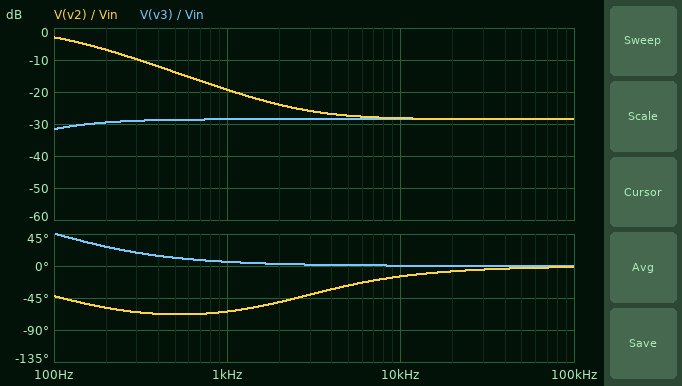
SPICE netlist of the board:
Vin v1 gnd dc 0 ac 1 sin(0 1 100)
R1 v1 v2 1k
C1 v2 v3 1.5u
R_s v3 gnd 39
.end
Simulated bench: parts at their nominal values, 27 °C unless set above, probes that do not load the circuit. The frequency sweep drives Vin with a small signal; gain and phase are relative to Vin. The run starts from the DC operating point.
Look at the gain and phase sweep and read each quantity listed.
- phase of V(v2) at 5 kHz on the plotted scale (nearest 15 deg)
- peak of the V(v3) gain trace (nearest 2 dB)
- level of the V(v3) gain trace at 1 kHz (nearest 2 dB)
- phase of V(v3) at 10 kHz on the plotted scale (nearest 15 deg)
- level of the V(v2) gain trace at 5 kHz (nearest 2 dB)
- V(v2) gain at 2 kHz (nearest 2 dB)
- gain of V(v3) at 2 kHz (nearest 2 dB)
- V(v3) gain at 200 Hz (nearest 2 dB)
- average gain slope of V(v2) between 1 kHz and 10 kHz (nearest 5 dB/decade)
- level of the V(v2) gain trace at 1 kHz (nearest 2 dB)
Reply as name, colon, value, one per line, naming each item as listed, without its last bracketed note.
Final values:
phase of V(v2) at 5 kHz on the plotted scale: -30 deg
peak of the V(v3) gain trace: -28 dB
level of the V(v3) gain trace at 1 kHz: -28 dB
phase of V(v3) at 10 kHz on the plotted scale: 0 deg
level of the V(v2) gain trace at 5 kHz: -28 dB
V(v2) gain at 2 kHz: -24 dB
gain of V(v3) at 2 kHz: -28 dB
V(v3) gain at 200 Hz: -30 dB
average gain slope of V(v2) between 1 kHz and 10 kHz: -10 dB/decade
level of the V(v2) gain trace at 1 kHz: -20 dB
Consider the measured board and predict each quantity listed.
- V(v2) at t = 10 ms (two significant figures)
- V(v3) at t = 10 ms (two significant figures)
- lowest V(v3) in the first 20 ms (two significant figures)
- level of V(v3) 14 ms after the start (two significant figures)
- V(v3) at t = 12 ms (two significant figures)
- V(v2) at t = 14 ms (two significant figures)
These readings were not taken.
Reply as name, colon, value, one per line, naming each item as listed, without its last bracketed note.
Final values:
V(v2) at t = 10 ms: -480 mV
V(v3) at t = 10 ms: 19 mV
lowest V(v3) in the first 20 ms: -27 mV
level of V(v3) 14 ms after the start: -4.4 mV
V(v3) at t = 12 ms: 23 mV
V(v2) at t = 14 ms: 700 mV
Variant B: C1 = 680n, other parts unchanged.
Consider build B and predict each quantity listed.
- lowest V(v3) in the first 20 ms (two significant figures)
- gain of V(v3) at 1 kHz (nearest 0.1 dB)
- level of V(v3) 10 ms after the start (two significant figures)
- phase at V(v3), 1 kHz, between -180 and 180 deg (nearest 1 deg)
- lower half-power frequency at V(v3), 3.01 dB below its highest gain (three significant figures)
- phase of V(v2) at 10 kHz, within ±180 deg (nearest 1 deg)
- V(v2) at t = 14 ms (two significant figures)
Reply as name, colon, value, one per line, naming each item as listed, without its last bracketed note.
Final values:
lowest V(v3) in the first 20 ms: -15 mV
gain of V(v3) at 1 kHz: -28.7 dB
level of V(v3) 10 ms after the start: 14 mV
phase at V(v3), 1 kHz, between -180 and 180 deg: 13 deg
lower half-power frequency at V(v3), 3.01 dB below its highest gain: 225 Hz
phase of V(v2) at 10 kHz, within ±180 deg: -30 deg
V(v2) at t = 14 ms: 780 mV
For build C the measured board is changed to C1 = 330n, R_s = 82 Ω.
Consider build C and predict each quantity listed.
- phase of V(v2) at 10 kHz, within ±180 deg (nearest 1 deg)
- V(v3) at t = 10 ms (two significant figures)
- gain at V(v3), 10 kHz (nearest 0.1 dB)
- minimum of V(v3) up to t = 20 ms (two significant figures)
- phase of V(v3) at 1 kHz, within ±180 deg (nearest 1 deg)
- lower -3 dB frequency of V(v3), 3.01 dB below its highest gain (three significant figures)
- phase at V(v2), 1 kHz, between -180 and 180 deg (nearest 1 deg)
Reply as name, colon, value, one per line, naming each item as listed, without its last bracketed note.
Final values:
phase of V(v2) at 10 kHz, within ±180 deg: -28 deg
V(v3) at t = 10 ms: 16 mV
gain at V(v3), 10 kHz: -22.4 dB
minimum of V(v3) up to t = 20 ms: -17 mV
phase of V(v3) at 1 kHz, within ±180 deg: 24 deg
lower -3 dB frequency of V(v3), 3.01 dB below its highest gain: 446 Hz
phase at V(v2), 1 kHz, between -180 and 180 deg: -56 deg
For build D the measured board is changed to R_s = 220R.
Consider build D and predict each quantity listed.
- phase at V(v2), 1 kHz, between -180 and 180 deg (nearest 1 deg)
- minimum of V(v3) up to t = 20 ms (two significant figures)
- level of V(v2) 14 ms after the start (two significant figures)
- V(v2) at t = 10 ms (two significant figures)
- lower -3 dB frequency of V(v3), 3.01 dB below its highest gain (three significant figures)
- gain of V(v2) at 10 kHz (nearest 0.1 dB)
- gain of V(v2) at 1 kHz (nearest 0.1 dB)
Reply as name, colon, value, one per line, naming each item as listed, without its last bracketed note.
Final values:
phase at V(v2), 1 kHz, between -180 and 180 deg: -21 deg
minimum of V(v3) up to t = 20 ms: -140 mV
level of V(v2) 14 ms after the start: 640 mV
V(v2) at t = 10 ms: -400 mV
lower -3 dB frequency of V(v3), 3.01 dB below its highest gain: 87.0 Hz
gain of V(v2) at 10 kHz: -14.9 dB
gain of V(v2) at 1 kHz: -14.0 dB
